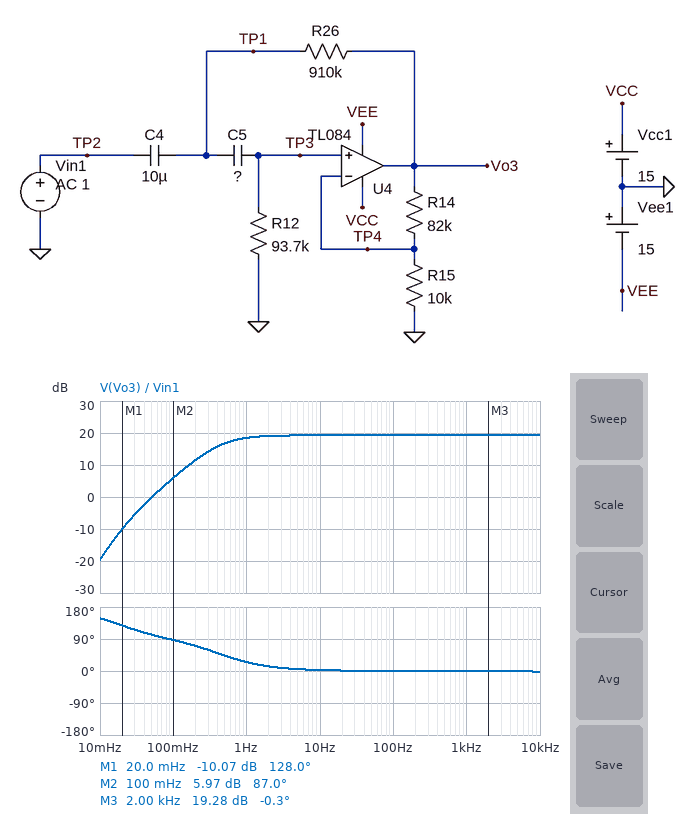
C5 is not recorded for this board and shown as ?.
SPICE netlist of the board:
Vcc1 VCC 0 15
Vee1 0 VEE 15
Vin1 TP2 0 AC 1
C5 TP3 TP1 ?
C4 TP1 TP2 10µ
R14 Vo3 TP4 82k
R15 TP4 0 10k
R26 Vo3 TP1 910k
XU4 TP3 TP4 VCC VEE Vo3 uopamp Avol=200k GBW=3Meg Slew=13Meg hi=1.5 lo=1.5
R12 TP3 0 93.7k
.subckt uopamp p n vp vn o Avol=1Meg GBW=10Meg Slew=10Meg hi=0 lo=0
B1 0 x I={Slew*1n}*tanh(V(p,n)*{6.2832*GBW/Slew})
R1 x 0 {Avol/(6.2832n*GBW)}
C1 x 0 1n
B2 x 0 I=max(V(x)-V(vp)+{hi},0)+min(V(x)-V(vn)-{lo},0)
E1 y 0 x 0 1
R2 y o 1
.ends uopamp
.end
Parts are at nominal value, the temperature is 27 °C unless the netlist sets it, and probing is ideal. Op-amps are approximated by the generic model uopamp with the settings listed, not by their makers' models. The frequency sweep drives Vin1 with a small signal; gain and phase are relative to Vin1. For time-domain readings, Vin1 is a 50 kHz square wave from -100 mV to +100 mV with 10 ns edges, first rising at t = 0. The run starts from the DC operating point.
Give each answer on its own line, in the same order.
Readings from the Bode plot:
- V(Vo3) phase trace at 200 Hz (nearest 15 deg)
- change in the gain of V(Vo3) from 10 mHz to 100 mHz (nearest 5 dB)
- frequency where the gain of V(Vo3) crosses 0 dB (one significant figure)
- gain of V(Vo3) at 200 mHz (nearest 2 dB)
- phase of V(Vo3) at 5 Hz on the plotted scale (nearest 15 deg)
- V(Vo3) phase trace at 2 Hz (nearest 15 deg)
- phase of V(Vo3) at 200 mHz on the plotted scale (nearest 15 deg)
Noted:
0 deg
25 dB
50 mHz
12 dB
0 deg
15 deg
75 deg
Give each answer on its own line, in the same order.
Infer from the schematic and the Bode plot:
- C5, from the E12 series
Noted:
3.9 µF
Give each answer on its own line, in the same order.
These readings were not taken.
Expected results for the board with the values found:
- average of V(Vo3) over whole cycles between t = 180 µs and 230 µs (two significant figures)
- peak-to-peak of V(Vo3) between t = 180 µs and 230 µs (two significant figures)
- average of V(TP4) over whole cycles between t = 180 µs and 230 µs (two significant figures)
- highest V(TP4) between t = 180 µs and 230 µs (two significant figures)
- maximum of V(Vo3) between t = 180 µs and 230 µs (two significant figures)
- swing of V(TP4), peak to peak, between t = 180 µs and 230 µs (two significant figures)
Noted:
920 mV
1.8 V
100 mV
200 mV
1.8 V
200 mV
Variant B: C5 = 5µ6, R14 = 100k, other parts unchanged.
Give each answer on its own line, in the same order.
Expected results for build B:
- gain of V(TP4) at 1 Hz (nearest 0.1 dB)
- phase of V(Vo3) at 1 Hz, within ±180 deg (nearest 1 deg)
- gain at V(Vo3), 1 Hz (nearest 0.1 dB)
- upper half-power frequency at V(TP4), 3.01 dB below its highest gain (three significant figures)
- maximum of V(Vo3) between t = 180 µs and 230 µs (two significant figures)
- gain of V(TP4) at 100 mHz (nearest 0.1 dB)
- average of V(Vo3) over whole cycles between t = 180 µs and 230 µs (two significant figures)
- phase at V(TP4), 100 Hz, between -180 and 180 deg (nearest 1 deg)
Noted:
-0.3 dB
17 deg
20.5 dB
273 kHz
2.2 V
-9.6 dB
1.1 V
0 deg
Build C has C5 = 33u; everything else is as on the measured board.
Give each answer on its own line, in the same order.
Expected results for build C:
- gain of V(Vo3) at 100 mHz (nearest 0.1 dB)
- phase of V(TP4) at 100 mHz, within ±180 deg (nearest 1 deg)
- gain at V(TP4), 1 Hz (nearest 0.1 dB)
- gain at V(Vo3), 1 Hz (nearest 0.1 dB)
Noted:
17.7 dB
41 deg
0 dB
19.3 dB
